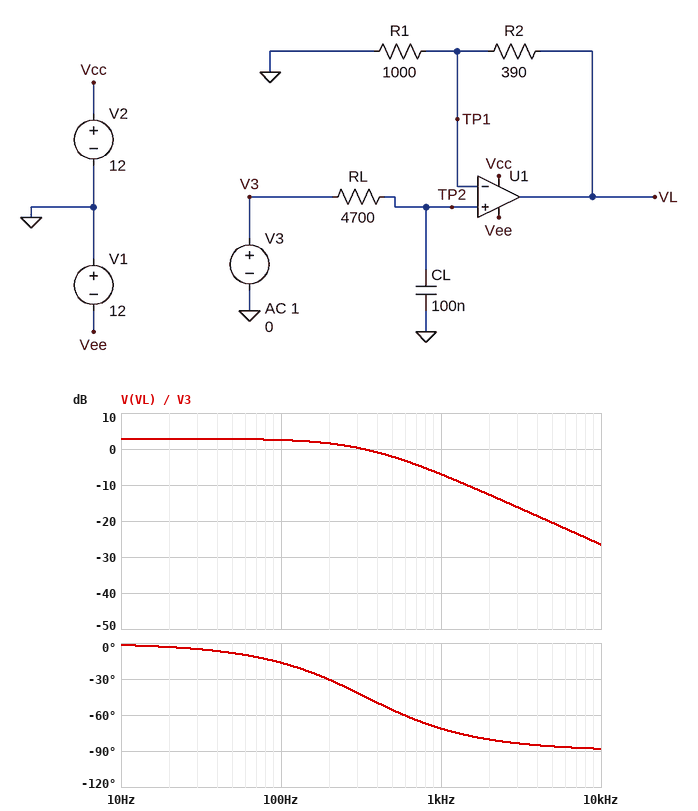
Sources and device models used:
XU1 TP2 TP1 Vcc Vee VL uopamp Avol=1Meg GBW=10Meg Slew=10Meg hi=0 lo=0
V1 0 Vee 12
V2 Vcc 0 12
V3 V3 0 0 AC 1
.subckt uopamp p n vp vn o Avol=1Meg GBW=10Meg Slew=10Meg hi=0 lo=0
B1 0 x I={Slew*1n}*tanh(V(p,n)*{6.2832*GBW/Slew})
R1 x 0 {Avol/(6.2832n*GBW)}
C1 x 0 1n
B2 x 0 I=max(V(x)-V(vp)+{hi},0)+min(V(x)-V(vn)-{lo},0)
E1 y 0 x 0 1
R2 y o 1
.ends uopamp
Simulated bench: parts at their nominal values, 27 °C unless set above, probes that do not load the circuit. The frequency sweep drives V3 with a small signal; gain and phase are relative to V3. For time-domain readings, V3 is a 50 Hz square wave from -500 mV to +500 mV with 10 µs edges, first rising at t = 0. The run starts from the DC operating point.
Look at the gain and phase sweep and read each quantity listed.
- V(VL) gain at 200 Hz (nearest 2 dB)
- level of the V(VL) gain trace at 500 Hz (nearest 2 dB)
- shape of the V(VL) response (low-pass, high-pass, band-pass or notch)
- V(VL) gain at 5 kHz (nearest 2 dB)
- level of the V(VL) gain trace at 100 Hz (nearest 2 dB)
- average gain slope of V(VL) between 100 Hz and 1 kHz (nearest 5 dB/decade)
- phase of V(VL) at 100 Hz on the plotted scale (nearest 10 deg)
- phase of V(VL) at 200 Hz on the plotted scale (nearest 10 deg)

2 dB
-2 dB
low-pass
-20 dB
2 dB
-10 dB/decade
-20 deg
-30 deg
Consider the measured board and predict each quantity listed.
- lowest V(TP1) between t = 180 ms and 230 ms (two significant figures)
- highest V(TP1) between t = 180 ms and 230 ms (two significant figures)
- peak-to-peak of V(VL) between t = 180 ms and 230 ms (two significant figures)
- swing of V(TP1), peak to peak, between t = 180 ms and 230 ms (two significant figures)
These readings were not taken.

-500 mV
500 mV
1.4 V
1.0 V
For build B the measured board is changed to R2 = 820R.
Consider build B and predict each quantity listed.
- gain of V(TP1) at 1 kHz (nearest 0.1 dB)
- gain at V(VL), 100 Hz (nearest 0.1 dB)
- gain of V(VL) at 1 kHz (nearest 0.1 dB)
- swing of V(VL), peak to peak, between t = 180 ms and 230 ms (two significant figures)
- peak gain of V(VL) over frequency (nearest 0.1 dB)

-9.9 dB
4.8 dB
-4.7 dB
1.8 V
5.2 dB
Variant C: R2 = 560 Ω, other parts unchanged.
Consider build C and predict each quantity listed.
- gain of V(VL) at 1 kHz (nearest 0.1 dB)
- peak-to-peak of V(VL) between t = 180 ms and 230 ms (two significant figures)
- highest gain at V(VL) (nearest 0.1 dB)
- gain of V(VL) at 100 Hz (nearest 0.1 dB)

-6.0 dB
1.6 V
3.9 dB
3.5 dB
